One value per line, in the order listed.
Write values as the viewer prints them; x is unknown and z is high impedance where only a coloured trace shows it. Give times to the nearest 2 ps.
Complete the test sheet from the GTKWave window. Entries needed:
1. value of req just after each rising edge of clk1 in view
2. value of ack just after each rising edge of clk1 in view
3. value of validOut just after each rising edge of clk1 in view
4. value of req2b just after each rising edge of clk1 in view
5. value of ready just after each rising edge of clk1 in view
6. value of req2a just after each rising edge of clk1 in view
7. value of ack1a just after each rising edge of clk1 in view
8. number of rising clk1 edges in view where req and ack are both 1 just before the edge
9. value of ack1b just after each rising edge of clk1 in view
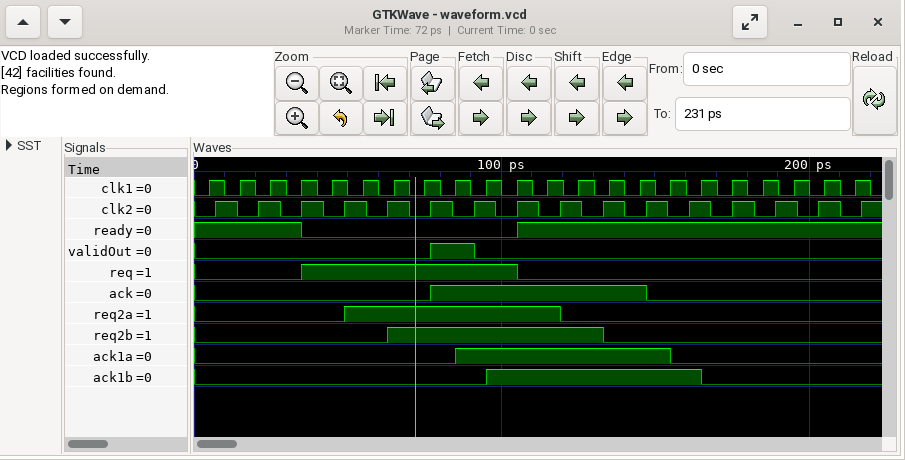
0 0 0 1 1 1 1 1 1 1 0 0 0 0 0 0 0 0 0 0 0 0
0 0 0 0 0 0 0 0 1 1 1 1 1 1 1 0 0 0 0 0 0 0
0 0 0 0 0 0 0 0 1 0 0 0 0 0 0 0 0 0 0 0 0 0
0 0 0 0 0 0 1 1 1 1 1 1 1 0 0 0 0 0 0 0 0 0
1 1 1 0 0 0 0 0 0 0 1 1 1 1 1 1 1 1 1 1 1 1
0 0 0 0 0 1 1 1 1 1 1 1 0 0 0 0 0 0 0 0 0 0
0 0 0 0 0 0 0 0 1 1 1 1 1 1 1 0 0 0 0 0 0 0
3
0 0 0 0 0 0 0 0 0 1 1 1 1 1 1 1 0 0 0 0 0 0
